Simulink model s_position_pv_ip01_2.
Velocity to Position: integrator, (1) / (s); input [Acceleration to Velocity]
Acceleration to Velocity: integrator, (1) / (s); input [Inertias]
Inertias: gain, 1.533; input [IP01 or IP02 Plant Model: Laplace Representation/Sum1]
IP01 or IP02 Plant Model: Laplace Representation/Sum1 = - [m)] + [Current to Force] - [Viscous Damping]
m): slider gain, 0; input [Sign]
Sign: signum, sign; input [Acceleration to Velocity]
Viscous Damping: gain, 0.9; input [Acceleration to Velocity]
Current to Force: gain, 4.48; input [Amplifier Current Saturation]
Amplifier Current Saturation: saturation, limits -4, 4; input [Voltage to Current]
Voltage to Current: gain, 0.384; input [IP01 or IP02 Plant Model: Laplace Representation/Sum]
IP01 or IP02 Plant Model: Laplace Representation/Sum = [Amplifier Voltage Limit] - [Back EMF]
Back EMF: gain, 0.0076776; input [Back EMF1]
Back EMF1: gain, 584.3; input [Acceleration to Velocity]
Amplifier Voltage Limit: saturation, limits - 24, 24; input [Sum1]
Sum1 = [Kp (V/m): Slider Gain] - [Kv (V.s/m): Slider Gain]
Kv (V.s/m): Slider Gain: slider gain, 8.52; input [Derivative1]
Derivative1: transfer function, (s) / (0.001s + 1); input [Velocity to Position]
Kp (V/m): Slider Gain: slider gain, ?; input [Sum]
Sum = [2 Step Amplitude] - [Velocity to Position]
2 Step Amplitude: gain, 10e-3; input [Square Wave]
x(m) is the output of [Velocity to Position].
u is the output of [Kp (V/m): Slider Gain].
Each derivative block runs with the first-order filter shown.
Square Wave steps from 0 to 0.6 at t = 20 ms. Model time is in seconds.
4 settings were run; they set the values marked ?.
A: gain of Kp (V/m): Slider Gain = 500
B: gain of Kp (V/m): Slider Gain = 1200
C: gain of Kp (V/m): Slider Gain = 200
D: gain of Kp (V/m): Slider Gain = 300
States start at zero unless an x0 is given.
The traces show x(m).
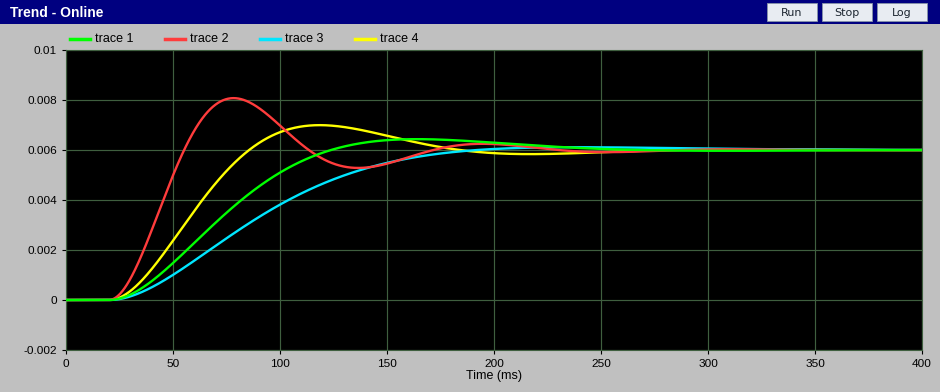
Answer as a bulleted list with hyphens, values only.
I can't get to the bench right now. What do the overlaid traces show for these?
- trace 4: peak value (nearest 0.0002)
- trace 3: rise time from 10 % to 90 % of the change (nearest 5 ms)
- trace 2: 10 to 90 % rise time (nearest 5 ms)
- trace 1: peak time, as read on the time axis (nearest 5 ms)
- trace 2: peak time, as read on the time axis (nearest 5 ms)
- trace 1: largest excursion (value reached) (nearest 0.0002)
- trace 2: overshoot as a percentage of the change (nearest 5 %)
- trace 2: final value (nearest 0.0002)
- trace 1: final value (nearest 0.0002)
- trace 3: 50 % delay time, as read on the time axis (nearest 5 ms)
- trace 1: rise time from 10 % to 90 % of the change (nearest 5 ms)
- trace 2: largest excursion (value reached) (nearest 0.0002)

- 0.0070
- 105 ms
- 25 ms
- 165 ms
- 80 ms
- 0.0064
- 35 %
- 0.0060
- 0.0060
- 85 ms
- 70 ms
- 0.0080
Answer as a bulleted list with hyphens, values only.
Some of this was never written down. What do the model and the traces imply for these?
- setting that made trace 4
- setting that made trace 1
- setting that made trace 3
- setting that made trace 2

- A
- D
- C
- B
